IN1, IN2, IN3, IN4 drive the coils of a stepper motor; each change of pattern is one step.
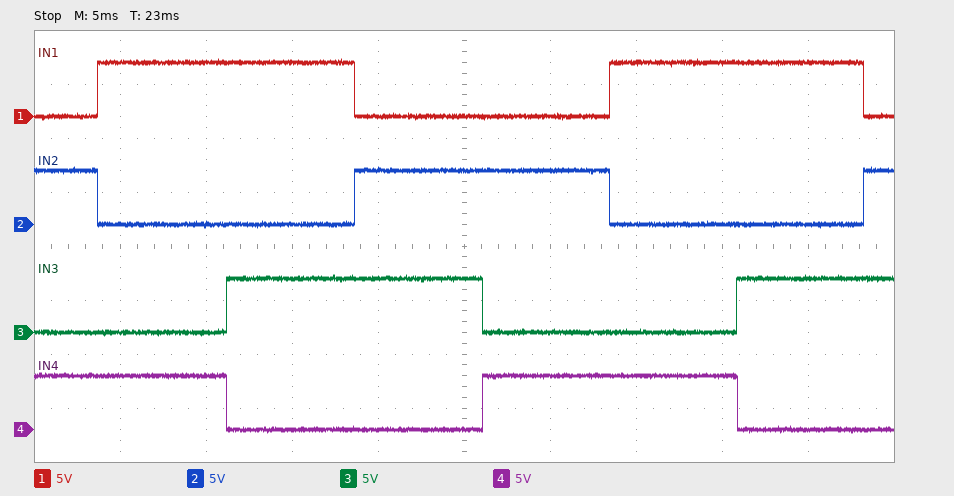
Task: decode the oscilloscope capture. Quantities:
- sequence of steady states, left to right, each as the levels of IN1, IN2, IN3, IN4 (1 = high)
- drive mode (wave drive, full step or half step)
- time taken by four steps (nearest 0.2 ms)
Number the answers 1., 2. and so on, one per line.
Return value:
1. 0101 1001 1010 0110 0101 1001 1010 0110
2. full step
3. 29.8 ms
